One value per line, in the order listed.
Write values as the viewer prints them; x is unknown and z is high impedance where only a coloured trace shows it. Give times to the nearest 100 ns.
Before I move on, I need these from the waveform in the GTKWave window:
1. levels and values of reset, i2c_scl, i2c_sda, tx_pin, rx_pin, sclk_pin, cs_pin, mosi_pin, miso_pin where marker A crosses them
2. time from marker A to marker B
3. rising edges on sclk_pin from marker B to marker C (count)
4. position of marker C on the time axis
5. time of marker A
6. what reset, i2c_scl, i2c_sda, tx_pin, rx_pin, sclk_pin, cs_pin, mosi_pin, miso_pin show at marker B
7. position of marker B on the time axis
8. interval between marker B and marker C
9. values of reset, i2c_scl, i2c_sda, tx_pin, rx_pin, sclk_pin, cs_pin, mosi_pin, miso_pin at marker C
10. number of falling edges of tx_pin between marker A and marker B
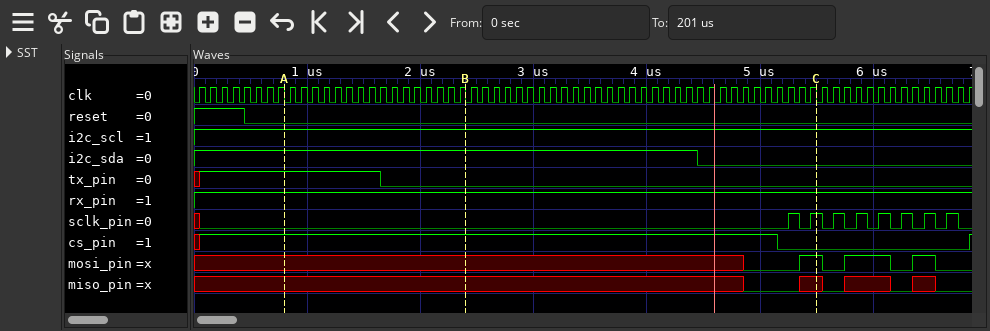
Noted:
reset=0, i2c_scl=1, i2c_sda=1, tx_pin=1, rx_pin=1, sclk_pin=0, cs_pin=1, mosi_pin=x, miso_pin=x
1600 ns
2
5500 ns
800 ns
reset=0, i2c_scl=1, i2c_sda=1, tx_pin=0, rx_pin=1, sclk_pin=0, cs_pin=1, mosi_pin=x, miso_pin=x
2400 ns
3100 ns
reset=0, i2c_scl=1, i2c_sda=0, tx_pin=0, rx_pin=1, sclk_pin=1, cs_pin=0, mosi_pin=1, miso_pin=x
1
